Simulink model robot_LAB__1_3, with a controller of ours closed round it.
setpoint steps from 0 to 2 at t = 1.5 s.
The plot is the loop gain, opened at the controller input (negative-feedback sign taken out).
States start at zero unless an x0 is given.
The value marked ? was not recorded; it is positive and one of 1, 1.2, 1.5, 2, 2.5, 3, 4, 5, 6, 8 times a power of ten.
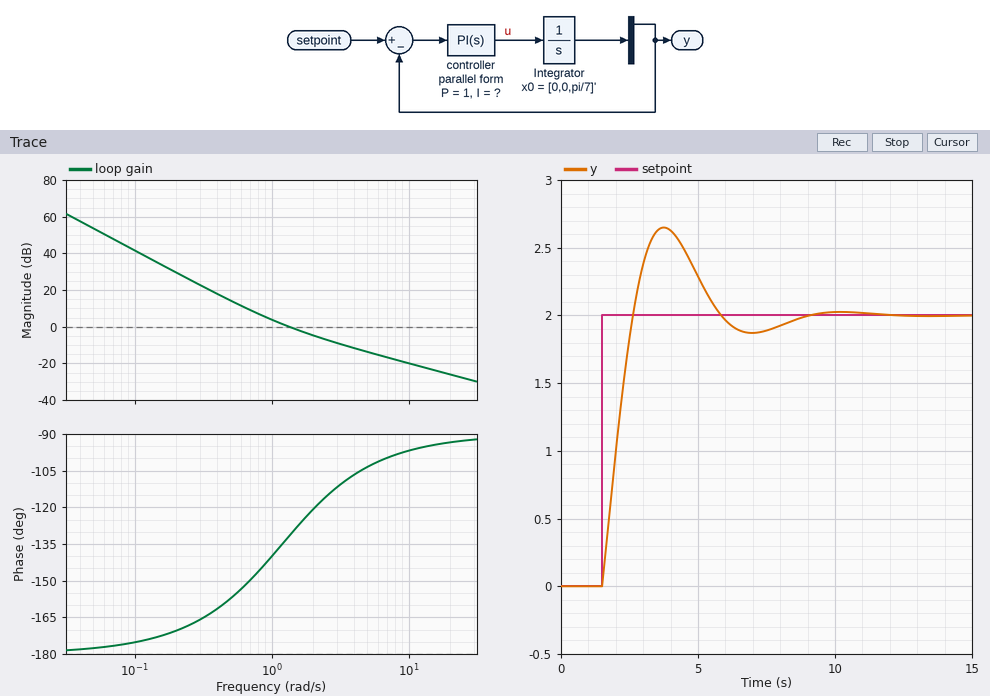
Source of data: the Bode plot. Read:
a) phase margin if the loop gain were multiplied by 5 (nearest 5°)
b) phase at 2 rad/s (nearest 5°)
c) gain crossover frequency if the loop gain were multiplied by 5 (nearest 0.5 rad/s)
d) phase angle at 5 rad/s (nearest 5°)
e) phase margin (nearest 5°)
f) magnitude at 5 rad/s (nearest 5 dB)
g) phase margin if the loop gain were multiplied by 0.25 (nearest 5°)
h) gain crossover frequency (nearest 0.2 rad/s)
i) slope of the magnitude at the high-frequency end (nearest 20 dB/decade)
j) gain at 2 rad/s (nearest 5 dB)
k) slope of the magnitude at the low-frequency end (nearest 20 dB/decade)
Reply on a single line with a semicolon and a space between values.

75°; -120°; 5.0 rad/s; -105°; 50°; -15 dB; 25°; 1.4 rad/s; -20 dB/decade; -5 dB; -40 dB/decade
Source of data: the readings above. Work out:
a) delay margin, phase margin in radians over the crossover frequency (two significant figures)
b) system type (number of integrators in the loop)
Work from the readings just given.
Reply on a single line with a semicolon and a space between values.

0.62 s; 2
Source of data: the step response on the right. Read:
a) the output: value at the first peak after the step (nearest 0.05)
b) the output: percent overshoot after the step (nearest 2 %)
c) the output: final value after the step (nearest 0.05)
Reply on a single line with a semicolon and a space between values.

2.65; 32 %; 2.00
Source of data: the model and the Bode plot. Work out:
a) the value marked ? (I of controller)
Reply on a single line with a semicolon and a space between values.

1.2
